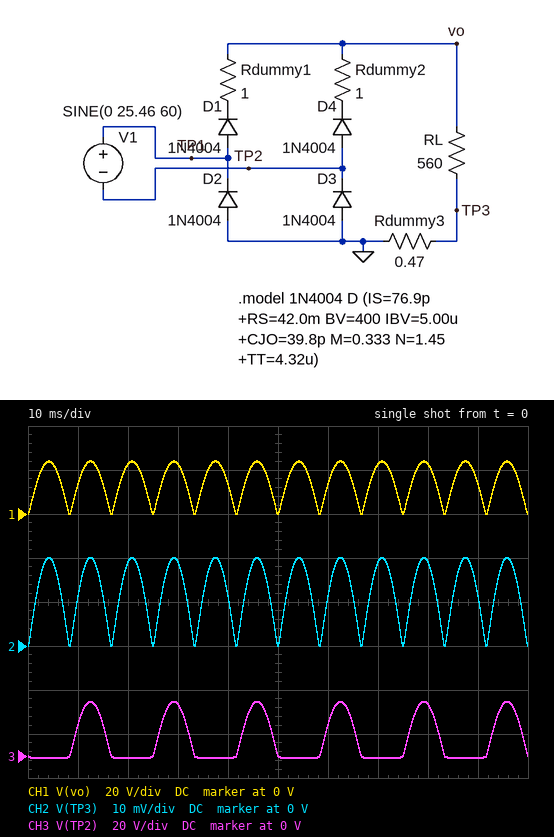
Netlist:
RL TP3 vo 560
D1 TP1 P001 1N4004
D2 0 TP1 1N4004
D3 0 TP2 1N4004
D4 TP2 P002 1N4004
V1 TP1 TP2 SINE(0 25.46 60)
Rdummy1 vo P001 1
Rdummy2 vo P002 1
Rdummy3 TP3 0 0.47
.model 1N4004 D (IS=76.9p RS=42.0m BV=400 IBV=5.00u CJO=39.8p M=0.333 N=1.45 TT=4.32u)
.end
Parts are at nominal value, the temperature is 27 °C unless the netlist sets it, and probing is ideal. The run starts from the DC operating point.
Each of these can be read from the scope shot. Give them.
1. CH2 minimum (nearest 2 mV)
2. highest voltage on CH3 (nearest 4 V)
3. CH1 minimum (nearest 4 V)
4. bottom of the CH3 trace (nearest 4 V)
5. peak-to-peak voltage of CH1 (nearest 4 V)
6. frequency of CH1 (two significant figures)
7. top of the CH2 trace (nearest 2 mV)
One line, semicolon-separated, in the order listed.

0 V; 24 V; 0 V; 0 V; 24 V; 120 Hz; 20 mV
